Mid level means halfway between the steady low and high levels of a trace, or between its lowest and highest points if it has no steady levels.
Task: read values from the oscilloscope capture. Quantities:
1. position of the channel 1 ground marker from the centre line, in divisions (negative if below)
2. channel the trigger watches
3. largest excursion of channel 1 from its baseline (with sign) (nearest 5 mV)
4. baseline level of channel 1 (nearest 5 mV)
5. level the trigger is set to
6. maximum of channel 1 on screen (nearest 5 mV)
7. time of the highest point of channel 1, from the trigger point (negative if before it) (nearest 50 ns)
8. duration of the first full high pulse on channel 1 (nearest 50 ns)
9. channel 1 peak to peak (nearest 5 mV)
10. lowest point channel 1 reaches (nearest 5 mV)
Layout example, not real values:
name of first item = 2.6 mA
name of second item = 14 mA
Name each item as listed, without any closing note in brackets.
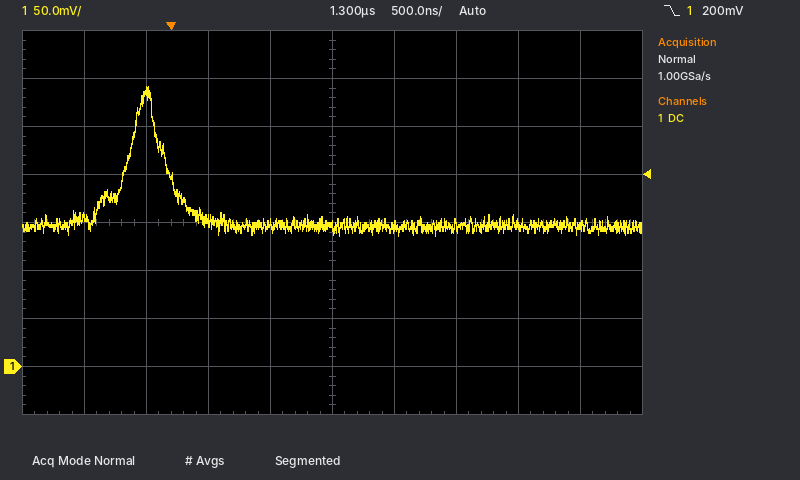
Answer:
position of the channel 1 ground marker from the centre line, in divisions = -3.0 div
channel the trigger watches = channel 1
largest excursion of channel 1 from its baseline (with sign) = +145 mV
baseline level of channel 1 = 145 mV
level the trigger is set to = 200 mV
maximum of channel 1 on screen = 290 mV
time of the highest point of channel 1, from the trigger point (negative if before it) = -200 ns
duration of the first full high pulse on channel 1 = 300 ns
channel 1 peak to peak = 155 mV
lowest point channel 1 reaches = 135 mV
